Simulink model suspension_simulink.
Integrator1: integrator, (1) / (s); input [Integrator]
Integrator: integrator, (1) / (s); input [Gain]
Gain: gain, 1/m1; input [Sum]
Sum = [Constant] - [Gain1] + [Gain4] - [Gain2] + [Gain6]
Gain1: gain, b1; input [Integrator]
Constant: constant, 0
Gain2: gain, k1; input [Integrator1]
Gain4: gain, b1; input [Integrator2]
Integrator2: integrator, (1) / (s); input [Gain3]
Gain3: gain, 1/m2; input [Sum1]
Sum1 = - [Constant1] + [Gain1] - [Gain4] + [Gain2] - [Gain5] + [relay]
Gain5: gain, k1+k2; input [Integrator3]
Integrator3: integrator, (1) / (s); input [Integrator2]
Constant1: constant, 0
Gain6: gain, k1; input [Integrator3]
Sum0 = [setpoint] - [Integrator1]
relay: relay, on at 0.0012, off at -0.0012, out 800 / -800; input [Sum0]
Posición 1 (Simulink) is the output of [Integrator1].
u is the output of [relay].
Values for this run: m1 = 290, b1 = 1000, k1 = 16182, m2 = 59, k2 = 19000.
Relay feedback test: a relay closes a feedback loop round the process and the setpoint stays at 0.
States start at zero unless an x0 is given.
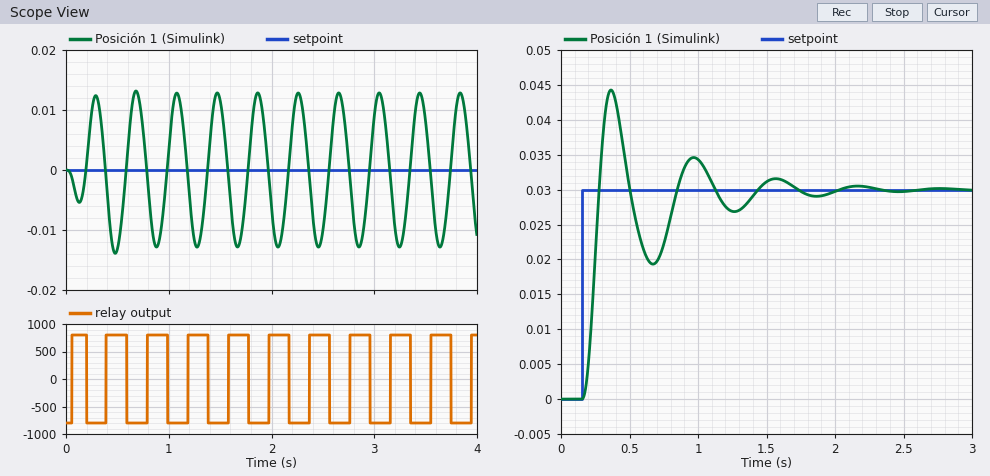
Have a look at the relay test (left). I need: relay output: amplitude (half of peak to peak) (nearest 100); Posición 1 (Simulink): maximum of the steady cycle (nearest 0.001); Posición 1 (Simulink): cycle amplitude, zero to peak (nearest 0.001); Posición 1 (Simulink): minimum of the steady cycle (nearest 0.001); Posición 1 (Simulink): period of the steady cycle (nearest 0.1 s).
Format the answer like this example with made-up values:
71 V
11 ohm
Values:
800
0.013
0.013
-0.013
0.4 s
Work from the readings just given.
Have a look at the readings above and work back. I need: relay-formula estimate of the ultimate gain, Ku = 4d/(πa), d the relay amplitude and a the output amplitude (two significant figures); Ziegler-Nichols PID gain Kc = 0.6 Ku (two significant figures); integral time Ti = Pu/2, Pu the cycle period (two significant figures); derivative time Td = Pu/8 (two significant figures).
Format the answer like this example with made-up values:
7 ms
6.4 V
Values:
78000
47000
0.20 s
0.050 s
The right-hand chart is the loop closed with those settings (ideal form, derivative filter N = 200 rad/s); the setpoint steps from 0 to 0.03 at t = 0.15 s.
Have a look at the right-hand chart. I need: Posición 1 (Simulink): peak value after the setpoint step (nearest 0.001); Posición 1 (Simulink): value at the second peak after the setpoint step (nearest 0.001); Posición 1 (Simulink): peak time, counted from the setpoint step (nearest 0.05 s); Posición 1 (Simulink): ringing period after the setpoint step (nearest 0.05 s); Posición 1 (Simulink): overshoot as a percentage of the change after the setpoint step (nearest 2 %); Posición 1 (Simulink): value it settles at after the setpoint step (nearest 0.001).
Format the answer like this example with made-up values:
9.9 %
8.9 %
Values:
0.044
0.035
0.20 s
0.60 s
48 %
0.030
